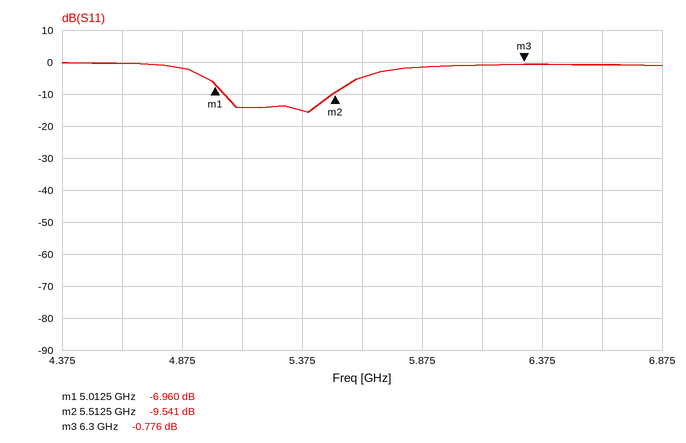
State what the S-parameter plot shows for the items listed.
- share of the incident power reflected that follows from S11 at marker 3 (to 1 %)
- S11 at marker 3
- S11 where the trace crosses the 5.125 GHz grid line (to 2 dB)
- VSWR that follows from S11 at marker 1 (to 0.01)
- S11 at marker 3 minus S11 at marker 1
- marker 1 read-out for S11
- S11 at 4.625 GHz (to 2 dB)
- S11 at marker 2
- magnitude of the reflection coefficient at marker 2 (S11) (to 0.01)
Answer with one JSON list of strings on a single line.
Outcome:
["84 %", "-0.776 dB", "-14 dB", "2.63", "6.184 dB", "-6.960 dB", "0 dB", "-9.541 dB", "0.33"]
